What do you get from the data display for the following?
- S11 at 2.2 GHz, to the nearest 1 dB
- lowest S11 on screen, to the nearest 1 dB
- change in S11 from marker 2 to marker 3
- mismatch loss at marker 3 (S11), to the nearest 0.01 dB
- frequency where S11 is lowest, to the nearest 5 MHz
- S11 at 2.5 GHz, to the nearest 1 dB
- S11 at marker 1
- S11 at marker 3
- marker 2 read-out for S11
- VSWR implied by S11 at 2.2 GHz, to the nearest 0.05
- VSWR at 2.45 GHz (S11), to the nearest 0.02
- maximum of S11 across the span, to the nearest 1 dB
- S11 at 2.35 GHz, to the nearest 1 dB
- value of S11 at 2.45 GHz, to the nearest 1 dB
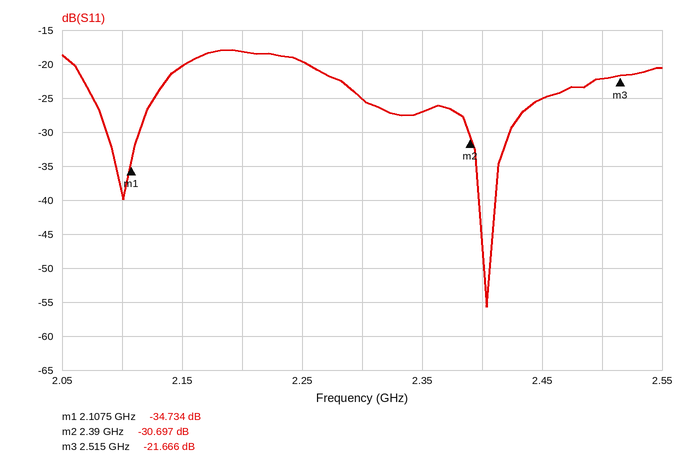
-18 dB
-56 dB
9.031 dB
0.03 dB
2.405 GHz
-22 dB
-34.734 dB
-21.666 dB
-30.697 dB
1.30
1.12
-18 dB
-27 dB
-25 dB
